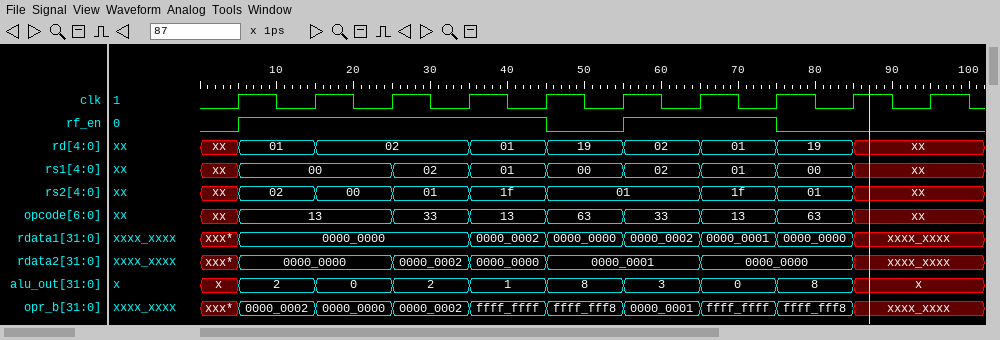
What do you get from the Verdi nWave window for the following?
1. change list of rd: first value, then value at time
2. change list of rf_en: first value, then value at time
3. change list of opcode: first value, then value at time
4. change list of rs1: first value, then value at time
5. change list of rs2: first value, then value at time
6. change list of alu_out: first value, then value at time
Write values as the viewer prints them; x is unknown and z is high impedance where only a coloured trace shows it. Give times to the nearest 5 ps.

xx, 01 at 5 ps, 02 at 15 ps, 01 at 35 ps, 19 at 45 ps, 02 at 55 ps, 01 at 65 ps, 19 at 75 ps, xx at 85 ps
0, 1 at 5 ps, 0 at 45 ps, 1 at 55 ps, 0 at 75 ps
xx, 13 at 5 ps, 33 at 25 ps, 13 at 35 ps, 63 at 45 ps, 33 at 55 ps, 13 at 65 ps, 63 at 75 ps, xx at 85 ps
xx, 00 at 5 ps, 02 at 25 ps, 01 at 35 ps, 00 at 45 ps, 02 at 55 ps, 01 at 65 ps, 00 at 75 ps, xx at 85 ps
xx, 02 at 5 ps, 00 at 15 ps, 01 at 25 ps, 1f at 35 ps, 01 at 45 ps, 1f at 65 ps, 01 at 75 ps, xx at 85 ps
x, 2 at 5 ps, 0 at 15 ps, 2 at 25 ps, 1 at 35 ps, 8 at 45 ps, 3 at 55 ps, 0 at 65 ps, 8 at 75 ps, x at 85 ps
